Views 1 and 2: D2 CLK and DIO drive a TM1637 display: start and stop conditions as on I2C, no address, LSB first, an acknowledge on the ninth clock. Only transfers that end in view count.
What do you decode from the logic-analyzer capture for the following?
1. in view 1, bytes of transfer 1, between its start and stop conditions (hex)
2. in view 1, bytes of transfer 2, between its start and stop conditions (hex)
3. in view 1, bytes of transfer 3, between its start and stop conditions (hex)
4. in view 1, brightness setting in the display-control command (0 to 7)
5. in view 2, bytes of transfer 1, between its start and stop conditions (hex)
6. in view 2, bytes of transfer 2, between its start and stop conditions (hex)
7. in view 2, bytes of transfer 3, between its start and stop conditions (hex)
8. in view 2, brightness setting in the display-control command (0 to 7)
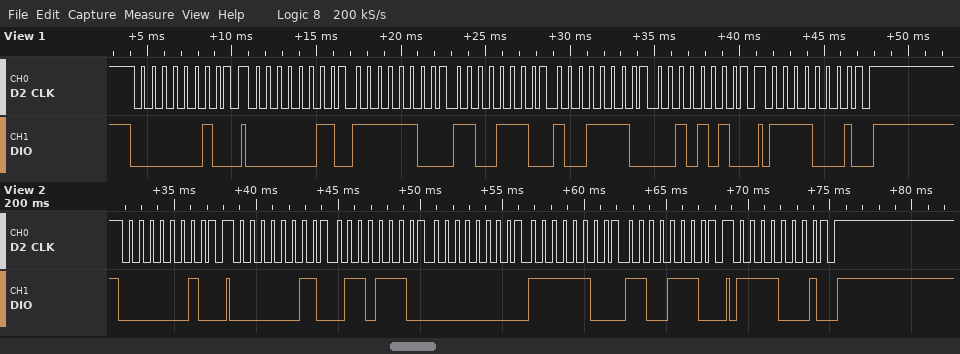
40
C0 3F 73 79 54
8F
7
40
C0 76 00 3F 73
8F
7
